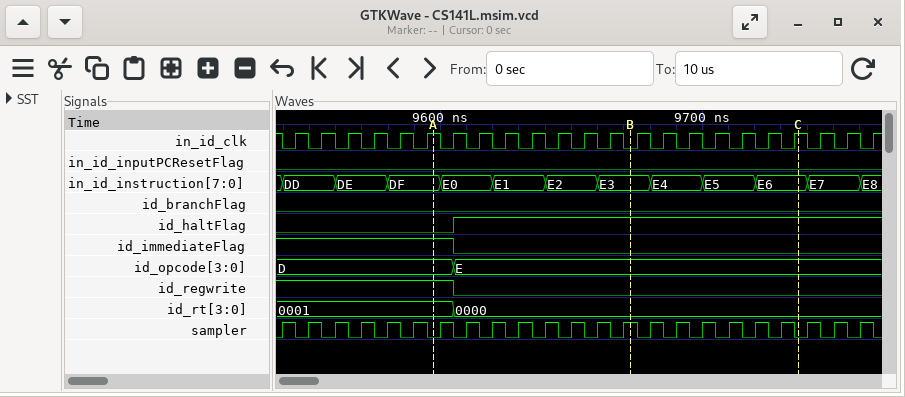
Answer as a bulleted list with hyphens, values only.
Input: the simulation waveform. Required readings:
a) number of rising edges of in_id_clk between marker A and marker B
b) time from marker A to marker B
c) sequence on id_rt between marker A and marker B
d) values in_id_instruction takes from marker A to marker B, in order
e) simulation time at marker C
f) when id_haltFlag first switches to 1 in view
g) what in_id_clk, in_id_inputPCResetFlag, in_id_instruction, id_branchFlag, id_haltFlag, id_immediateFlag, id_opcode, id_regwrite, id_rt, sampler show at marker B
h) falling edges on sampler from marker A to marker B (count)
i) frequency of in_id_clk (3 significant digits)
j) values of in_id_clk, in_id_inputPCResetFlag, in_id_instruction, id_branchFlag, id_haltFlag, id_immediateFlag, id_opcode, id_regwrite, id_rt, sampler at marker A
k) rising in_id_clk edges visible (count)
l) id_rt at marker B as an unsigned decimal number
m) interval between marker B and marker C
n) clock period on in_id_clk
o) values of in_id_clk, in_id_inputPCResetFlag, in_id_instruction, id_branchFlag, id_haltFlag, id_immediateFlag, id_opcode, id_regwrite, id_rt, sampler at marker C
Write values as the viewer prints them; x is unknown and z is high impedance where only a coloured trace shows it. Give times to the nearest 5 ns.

- 7
- 75 ns
- 0001, 0000
- DF, E0, E1, E2, E3
- 9735 ns
- 9605 ns
- in_id_clk=0, in_id_inputPCResetFlag=0, in_id_instruction=E3, id_branchFlag=0, id_haltFlag=1, id_immediateFlag=0, id_opcode=E, id_regwrite=0, id_rt=0000, sampler=1
- 7
- 100 MHz
- in_id_clk=1, in_id_inputPCResetFlag=0, in_id_instruction=DF, id_branchFlag=0, id_haltFlag=0, id_immediateFlag=1, id_opcode=D, id_regwrite=1, id_rt=0001, sampler=0
- 23
- 0
- 65 ns
- 10 ns
- in_id_clk=1, in_id_inputPCResetFlag=0, in_id_instruction=E6, id_branchFlag=0, id_haltFlag=1, id_immediateFlag=0, id_opcode=E, id_regwrite=0, id_rt=0000, sampler=0
